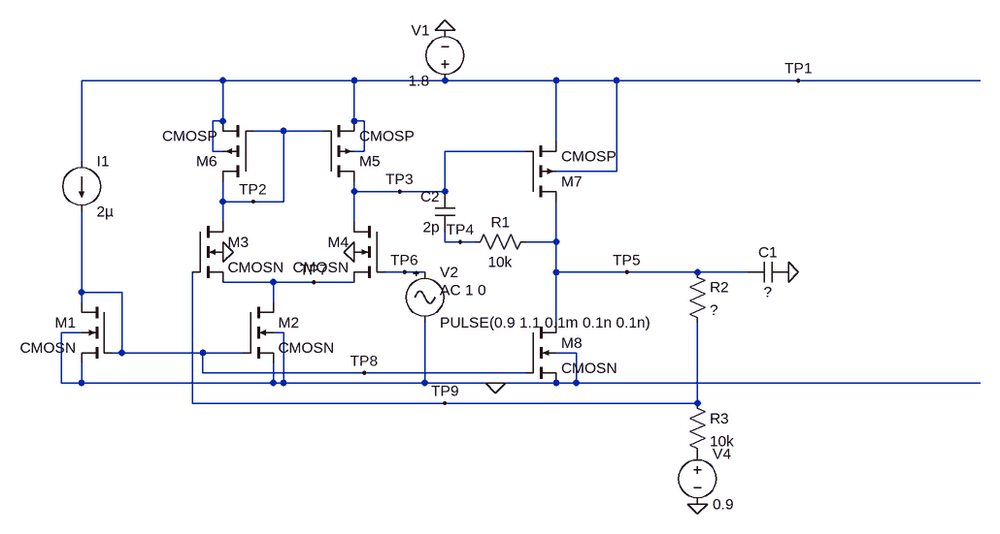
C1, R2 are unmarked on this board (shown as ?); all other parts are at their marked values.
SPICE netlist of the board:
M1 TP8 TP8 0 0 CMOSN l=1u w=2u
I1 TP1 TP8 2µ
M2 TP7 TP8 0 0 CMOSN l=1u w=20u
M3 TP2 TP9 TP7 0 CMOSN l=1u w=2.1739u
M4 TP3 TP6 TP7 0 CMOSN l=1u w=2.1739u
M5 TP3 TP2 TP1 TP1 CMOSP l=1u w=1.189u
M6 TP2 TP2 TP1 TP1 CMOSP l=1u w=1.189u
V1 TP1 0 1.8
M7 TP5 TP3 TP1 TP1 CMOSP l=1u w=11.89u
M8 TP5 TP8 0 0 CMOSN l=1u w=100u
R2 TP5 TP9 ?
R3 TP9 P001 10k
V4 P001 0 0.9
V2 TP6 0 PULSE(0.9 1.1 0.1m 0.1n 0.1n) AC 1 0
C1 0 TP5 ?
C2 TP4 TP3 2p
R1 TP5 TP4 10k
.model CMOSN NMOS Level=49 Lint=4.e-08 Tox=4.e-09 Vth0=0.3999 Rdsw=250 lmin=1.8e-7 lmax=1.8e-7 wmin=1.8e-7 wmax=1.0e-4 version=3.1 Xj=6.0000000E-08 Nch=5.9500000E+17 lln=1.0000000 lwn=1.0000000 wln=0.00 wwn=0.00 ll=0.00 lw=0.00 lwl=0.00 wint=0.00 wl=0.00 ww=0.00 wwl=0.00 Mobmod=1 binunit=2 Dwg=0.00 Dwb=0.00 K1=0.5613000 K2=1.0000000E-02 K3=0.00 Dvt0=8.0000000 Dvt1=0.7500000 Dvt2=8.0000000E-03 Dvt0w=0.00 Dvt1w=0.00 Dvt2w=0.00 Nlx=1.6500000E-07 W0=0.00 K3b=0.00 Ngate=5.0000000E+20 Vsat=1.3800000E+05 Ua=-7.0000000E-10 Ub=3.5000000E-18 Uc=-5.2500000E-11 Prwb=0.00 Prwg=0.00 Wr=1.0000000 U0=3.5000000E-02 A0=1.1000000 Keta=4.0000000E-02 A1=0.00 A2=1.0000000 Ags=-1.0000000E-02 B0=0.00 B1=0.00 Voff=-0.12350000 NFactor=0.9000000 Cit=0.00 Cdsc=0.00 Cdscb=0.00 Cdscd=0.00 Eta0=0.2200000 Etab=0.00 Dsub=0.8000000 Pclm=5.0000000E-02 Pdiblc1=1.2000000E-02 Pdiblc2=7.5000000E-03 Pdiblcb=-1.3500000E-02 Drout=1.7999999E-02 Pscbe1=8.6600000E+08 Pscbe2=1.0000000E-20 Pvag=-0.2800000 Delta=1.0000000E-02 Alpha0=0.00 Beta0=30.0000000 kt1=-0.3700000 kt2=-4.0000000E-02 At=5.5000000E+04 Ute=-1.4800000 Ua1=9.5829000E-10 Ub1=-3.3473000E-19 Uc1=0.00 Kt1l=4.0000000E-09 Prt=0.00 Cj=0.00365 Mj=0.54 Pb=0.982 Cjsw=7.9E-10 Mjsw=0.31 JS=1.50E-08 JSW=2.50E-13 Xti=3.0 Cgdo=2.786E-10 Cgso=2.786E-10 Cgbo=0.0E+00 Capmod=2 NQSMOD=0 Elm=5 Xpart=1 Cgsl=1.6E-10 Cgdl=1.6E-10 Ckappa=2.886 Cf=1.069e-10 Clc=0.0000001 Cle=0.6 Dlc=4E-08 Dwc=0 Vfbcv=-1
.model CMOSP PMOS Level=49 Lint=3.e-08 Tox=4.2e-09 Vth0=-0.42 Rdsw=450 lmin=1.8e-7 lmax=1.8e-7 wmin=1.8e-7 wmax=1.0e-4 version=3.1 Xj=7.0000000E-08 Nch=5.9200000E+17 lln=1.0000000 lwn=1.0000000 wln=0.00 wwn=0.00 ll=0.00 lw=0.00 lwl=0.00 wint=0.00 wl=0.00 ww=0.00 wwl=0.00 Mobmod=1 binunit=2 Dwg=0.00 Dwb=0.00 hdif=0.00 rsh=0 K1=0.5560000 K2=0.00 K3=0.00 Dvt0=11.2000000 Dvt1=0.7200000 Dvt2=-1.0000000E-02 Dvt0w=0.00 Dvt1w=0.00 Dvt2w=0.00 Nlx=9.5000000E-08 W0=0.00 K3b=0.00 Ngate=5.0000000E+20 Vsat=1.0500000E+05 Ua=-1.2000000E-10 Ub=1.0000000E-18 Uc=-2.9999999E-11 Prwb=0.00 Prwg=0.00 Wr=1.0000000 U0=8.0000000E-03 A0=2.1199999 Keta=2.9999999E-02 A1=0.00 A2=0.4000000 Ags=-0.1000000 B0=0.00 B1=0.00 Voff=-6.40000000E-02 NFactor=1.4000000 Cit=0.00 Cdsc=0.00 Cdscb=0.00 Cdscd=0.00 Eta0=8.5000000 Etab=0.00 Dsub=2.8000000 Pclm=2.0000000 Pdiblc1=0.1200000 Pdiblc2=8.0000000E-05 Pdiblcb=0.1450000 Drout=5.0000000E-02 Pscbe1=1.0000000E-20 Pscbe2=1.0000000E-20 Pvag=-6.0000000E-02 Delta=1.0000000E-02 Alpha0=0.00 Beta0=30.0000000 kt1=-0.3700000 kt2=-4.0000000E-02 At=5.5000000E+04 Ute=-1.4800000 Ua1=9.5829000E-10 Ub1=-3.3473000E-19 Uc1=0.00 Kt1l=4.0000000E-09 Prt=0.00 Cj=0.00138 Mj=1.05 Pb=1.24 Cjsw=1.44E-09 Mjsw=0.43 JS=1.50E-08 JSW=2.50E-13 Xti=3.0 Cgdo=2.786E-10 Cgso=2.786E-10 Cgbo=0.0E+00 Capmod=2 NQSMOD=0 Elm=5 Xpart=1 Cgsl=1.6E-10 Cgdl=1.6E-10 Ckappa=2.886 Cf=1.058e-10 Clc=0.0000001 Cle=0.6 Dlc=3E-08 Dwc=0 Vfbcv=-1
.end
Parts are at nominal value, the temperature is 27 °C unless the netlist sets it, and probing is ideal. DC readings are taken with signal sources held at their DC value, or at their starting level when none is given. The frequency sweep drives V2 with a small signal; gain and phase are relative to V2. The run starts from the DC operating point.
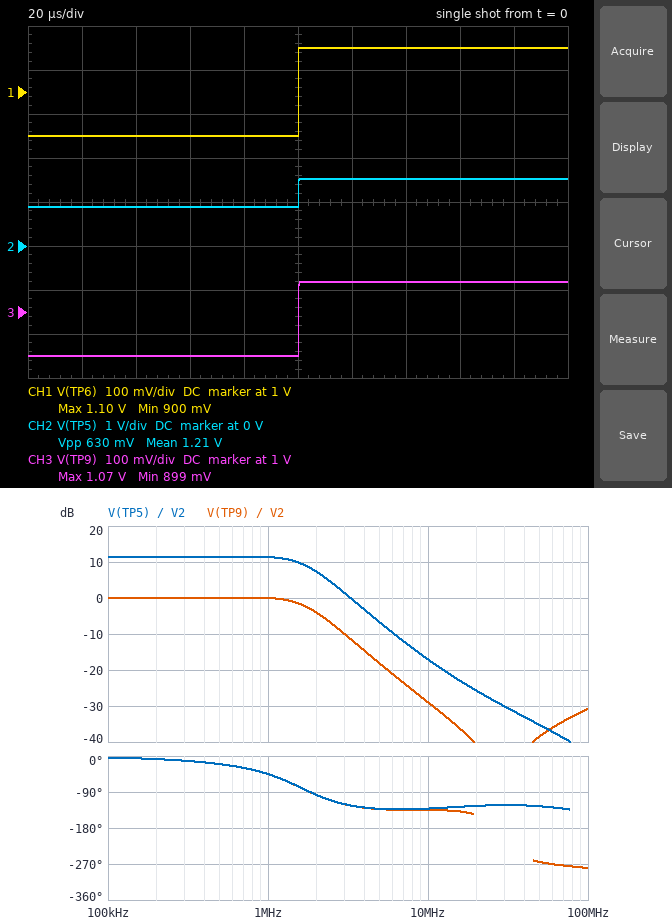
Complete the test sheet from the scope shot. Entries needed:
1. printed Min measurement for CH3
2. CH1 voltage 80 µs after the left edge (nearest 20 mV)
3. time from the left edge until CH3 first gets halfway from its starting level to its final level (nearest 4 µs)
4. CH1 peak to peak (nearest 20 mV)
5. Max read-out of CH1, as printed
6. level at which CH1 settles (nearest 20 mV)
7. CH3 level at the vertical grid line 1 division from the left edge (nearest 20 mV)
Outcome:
899 mV
900 mV
100 µs
200 mV
1.10 V
1.10 V
900 mV
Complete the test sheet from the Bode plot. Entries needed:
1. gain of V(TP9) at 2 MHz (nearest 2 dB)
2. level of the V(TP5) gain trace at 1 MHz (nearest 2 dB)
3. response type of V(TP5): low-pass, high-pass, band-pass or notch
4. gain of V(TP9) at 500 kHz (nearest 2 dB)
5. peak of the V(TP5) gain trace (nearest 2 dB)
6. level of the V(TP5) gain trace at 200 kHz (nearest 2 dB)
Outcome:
-4 dB
12 dB
low-pass
0 dB
12 dB
12 dB
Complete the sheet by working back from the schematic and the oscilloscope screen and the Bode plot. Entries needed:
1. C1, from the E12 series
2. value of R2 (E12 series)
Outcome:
27 pF
27 kΩ
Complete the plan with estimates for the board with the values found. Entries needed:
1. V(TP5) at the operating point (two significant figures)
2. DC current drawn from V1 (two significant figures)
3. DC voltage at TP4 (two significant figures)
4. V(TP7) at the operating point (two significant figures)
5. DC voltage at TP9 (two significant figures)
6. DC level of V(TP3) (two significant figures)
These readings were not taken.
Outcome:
900 mV
130 µA
900 mV
220 mV
900 mV
720 mV
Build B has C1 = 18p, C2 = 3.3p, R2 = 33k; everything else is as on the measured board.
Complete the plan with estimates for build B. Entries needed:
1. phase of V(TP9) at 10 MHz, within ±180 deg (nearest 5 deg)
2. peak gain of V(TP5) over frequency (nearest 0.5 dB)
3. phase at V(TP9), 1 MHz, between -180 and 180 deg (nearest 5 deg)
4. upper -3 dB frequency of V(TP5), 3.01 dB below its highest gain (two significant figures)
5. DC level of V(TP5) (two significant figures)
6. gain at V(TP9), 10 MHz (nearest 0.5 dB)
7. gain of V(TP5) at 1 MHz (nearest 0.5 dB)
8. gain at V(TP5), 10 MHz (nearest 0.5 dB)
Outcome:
-115 deg
12.5 dB
-60 deg
970 kHz
900 mV
-29.5 dB
9.5 dB
-16.0 dB
